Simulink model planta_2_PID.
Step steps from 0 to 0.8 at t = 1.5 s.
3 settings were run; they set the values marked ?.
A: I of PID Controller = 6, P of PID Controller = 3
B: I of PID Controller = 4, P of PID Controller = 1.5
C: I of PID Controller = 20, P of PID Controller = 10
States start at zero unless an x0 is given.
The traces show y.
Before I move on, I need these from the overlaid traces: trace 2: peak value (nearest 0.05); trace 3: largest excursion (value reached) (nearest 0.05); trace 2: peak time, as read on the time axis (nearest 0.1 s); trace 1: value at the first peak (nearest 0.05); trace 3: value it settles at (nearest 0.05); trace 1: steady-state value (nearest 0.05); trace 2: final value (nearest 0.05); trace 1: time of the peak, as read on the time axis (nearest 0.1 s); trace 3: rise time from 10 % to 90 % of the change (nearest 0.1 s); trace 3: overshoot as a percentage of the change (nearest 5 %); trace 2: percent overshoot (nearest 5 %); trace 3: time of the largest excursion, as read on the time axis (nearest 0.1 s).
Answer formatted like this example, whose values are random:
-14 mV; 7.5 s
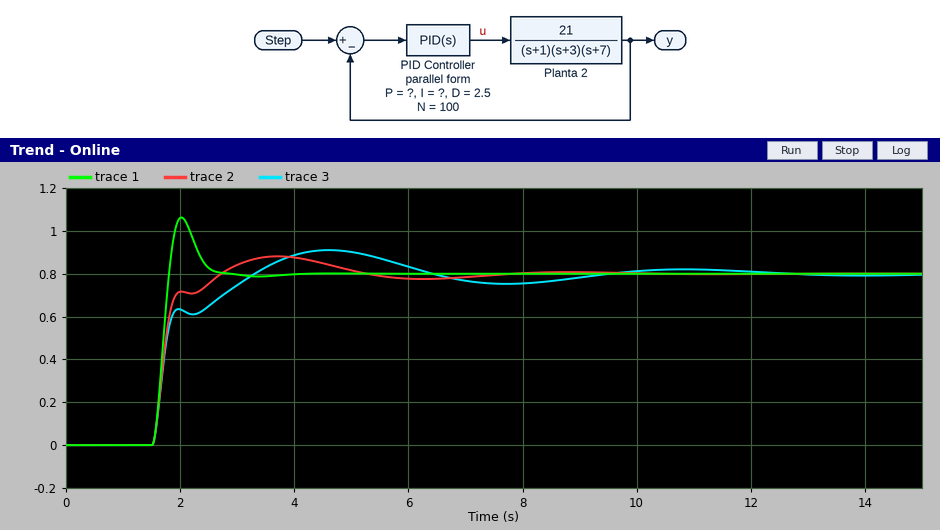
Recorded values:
0.90; 0.90; 3.7 s; 1.05; 0.80; 0.80; 0.80; 2.0 s; 1.3 s; 15 %; 10 %; 4.6 s
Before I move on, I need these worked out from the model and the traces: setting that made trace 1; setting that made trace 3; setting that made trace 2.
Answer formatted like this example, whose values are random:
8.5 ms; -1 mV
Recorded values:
C; B; A
